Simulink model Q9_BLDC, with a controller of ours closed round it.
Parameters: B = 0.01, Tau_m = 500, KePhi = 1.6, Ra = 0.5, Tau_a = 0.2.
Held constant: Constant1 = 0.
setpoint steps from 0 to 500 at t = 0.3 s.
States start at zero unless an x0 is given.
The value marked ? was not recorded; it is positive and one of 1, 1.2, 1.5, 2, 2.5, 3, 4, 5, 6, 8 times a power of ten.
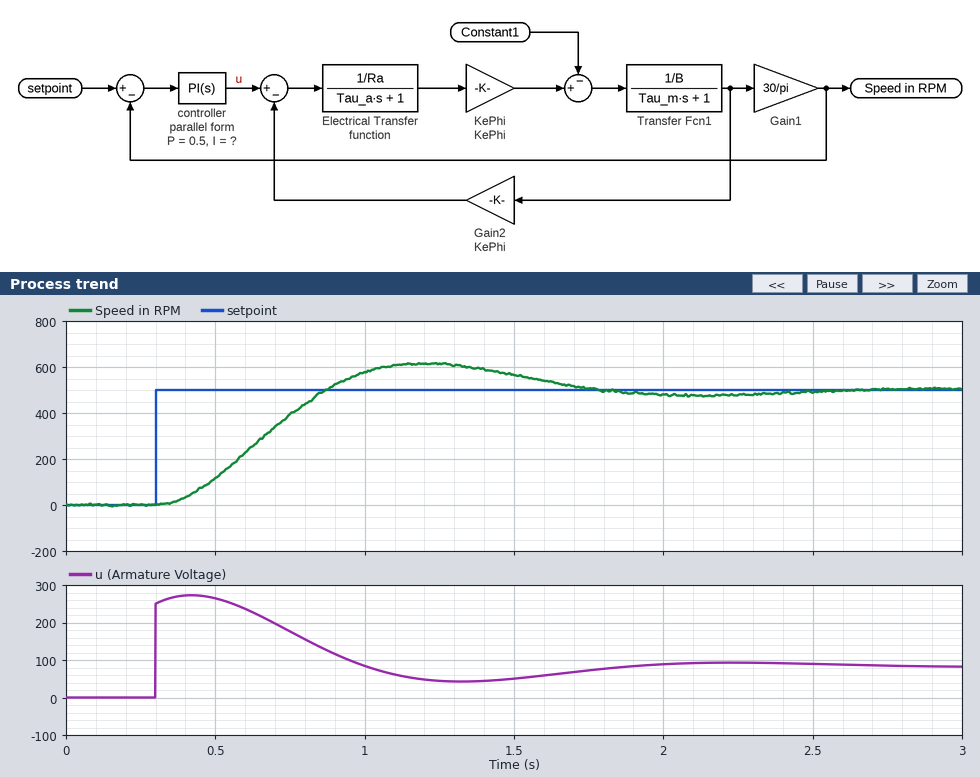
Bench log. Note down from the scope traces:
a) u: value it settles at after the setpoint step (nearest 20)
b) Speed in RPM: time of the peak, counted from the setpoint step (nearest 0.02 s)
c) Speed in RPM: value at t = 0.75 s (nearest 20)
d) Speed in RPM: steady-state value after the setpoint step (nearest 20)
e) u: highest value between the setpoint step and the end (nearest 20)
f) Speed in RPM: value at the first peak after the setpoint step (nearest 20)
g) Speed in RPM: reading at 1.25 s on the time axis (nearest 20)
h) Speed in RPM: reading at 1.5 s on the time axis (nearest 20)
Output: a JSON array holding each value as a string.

["80", "0.90 s", "400", "500", "280", "620", "620", "560"]
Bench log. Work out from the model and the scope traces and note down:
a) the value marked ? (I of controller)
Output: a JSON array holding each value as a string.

["0.8"]
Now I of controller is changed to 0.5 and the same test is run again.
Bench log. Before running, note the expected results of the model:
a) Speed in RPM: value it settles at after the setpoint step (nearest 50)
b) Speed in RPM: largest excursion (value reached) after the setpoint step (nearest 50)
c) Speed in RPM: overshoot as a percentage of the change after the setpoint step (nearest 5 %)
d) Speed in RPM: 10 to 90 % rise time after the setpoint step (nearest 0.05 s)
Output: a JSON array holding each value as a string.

["500", "550", "10 %", "0.45 s"]
